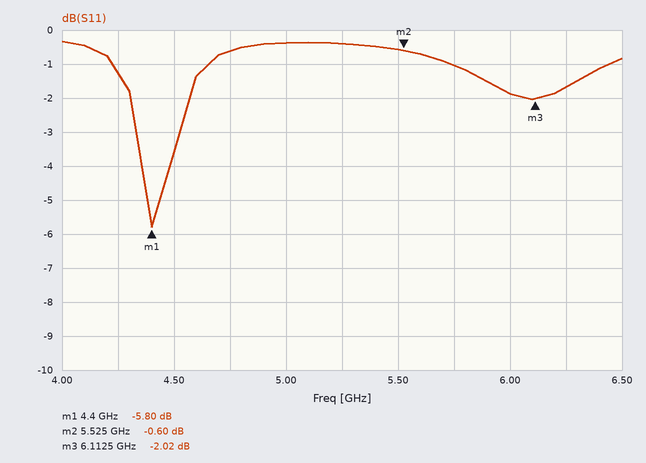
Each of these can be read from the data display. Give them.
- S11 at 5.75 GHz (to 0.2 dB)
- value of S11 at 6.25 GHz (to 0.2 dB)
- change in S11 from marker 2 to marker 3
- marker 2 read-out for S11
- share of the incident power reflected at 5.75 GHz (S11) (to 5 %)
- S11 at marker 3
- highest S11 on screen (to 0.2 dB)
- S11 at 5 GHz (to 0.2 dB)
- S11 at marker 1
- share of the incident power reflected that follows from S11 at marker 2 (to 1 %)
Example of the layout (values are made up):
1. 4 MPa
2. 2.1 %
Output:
1. -1.0 dB
2. -1.6 dB
3. -1.42 dB
4. -0.60 dB
5. 80 %
6. -2.02 dB
7. -0.4 dB
8. -0.4 dB
9. -5.80 dB
10. 87 %
